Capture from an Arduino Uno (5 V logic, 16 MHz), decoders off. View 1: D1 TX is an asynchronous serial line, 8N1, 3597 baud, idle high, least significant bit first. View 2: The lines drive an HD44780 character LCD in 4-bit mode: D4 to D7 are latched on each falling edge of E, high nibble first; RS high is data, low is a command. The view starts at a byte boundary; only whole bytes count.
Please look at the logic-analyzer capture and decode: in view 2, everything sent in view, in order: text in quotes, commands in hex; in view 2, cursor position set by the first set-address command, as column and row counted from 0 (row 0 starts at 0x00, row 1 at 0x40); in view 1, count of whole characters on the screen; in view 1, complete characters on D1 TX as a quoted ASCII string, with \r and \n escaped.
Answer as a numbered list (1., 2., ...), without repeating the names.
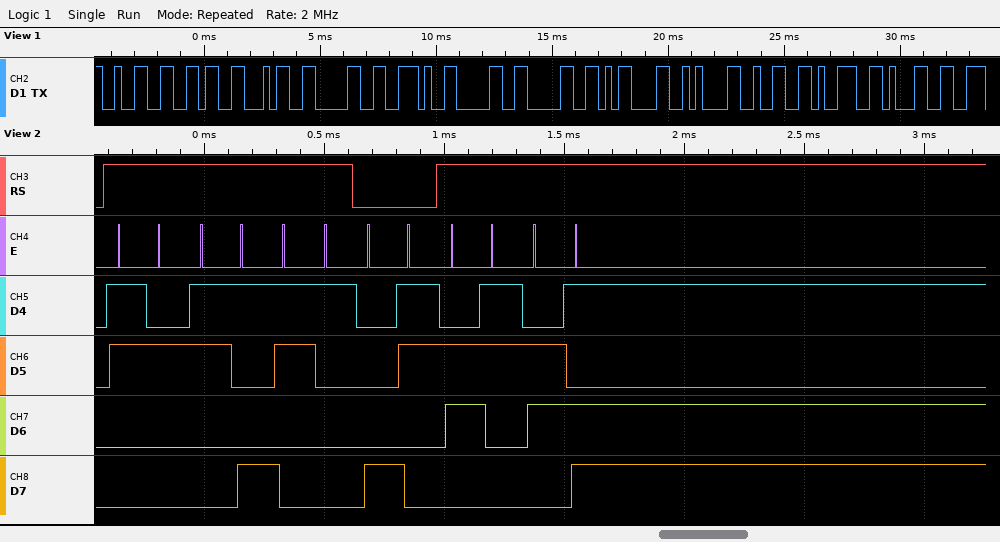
1. "291" 0x83 "cm"
2. column 3, row 0
3. 12
4. "2640.00\r\n291"
